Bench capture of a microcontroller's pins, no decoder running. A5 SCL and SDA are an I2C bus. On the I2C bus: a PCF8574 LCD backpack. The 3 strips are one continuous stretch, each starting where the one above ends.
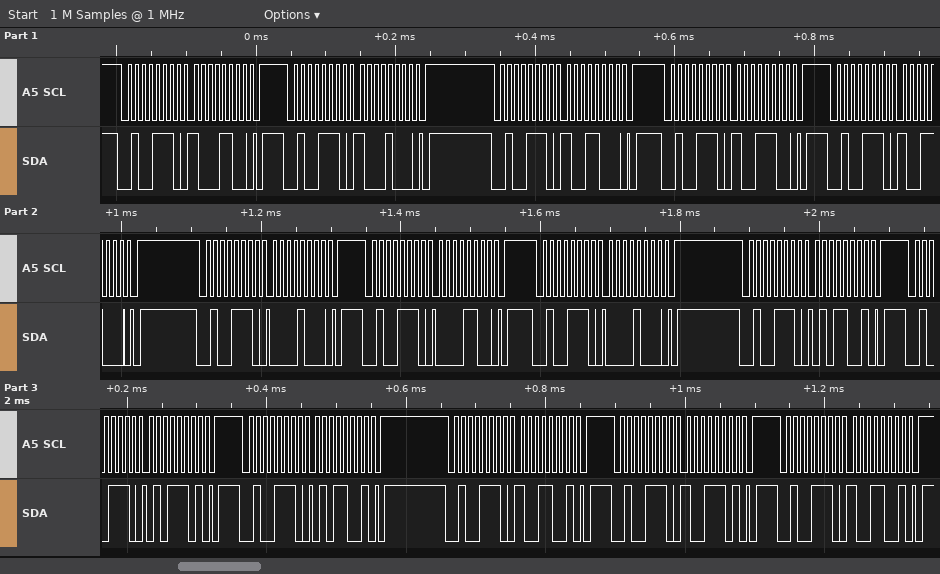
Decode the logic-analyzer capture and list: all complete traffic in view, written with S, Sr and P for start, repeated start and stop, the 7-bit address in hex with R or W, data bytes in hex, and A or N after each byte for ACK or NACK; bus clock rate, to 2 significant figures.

S 27W A 8C A P S 27W A 88 A P S 27W A 98 A P S 27W A 9C A P S 27W A 98 A P S 27W A 08 A P S 27W A 0C A P S 27W A 08 A P S 27W A 59 A P S 27W A 5D A P S 27W A 59 A P S 27W A 99 A P S 27W A 9D A P S 27W A 99 A P
100 kHz
